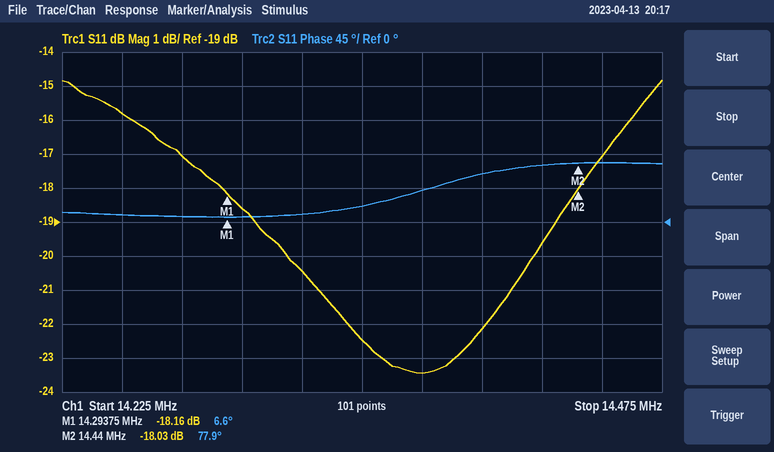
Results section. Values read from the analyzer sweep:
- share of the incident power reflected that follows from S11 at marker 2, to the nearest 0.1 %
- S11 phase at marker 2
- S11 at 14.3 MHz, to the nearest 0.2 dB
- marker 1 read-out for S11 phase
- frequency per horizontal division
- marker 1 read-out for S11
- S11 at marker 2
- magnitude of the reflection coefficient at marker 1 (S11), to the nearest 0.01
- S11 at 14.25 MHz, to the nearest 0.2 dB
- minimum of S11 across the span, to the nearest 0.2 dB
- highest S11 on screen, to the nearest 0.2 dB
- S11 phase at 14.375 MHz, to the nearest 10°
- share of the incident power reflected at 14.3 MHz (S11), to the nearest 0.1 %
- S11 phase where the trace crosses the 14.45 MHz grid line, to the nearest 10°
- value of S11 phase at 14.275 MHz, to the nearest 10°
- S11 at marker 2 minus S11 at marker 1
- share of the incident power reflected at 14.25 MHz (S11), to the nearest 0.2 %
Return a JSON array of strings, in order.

["1.6 %", "77.9°", "-18.6 dB", "6.6°", "25 kHz", "-18.16 dB", "-18.03 dB", "0.12", "-15.8 dB", "-23.4 dB", "-14.8 dB", "40°", "1.4 %", "80°", "10°", "0.13 dB", "2.6 %"]
